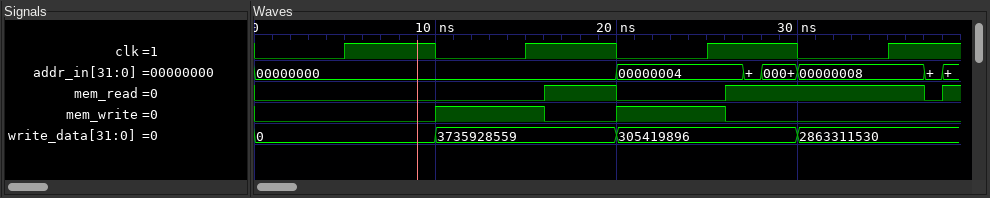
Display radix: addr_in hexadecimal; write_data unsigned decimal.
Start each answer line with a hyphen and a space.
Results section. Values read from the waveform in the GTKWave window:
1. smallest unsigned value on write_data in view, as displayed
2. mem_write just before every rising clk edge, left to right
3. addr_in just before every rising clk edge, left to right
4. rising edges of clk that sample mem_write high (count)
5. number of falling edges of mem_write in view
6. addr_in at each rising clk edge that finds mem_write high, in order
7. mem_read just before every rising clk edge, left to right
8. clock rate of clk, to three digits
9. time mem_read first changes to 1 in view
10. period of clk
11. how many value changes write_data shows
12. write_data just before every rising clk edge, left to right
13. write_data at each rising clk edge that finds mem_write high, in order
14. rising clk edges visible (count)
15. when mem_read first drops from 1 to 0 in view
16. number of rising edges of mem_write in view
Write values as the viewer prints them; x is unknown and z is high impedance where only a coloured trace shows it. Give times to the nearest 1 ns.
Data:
- 0
- 0 1 1 0
- 00000000, 00000000, 00000004, 00000008
- 2
- 2
- 00000000, 00000004
- 0 0 0 1
- 100 MHz
- 16 ns
- 10 ns
- 3
- 0, 3735928559, 305419896, 2863311530
- 3735928559, 305419896
- 4
- 20 ns
- 2
